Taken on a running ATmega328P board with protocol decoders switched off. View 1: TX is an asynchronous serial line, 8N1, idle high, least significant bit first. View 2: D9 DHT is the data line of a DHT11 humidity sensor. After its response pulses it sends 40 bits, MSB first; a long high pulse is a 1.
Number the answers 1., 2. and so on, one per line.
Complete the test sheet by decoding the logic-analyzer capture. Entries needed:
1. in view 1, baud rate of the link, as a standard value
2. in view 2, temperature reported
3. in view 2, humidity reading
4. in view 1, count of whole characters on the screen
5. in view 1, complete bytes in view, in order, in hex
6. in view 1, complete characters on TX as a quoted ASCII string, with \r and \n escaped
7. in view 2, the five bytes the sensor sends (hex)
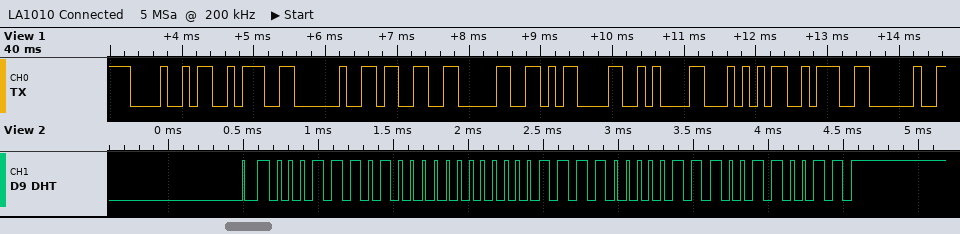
1. 9600 baud
2. 15.7 °C
3. 29 %
4. 10
5. 48 3A 20 33 30 0D 0A 54 3A 20
6. "H: 30\r\nT: "
7. 1D 00 0F 07 33
